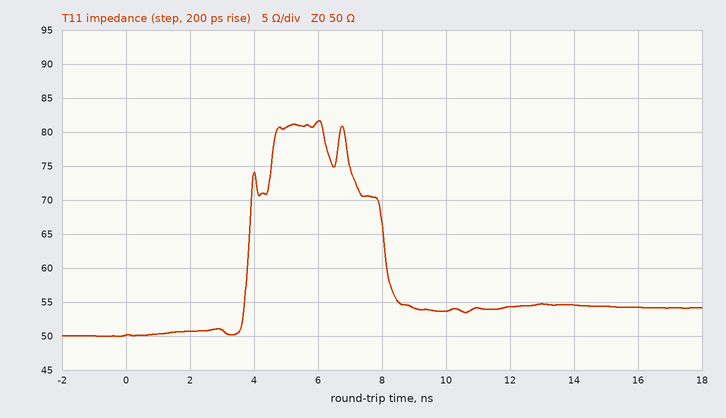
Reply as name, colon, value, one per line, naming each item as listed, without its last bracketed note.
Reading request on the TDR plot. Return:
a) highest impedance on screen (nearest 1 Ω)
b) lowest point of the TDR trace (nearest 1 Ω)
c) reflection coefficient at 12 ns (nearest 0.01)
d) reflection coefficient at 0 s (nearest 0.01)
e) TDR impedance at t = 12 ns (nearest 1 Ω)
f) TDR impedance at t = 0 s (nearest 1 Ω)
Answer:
highest impedance on screen: 82 Ω
lowest point of the TDR trace: 50 Ω
reflection coefficient at 12 ns: +0.04
reflection coefficient at 0 s: 0.00
TDR impedance at t = 12 ns: 54 Ω
TDR impedance at t = 0 s: 50 Ω
